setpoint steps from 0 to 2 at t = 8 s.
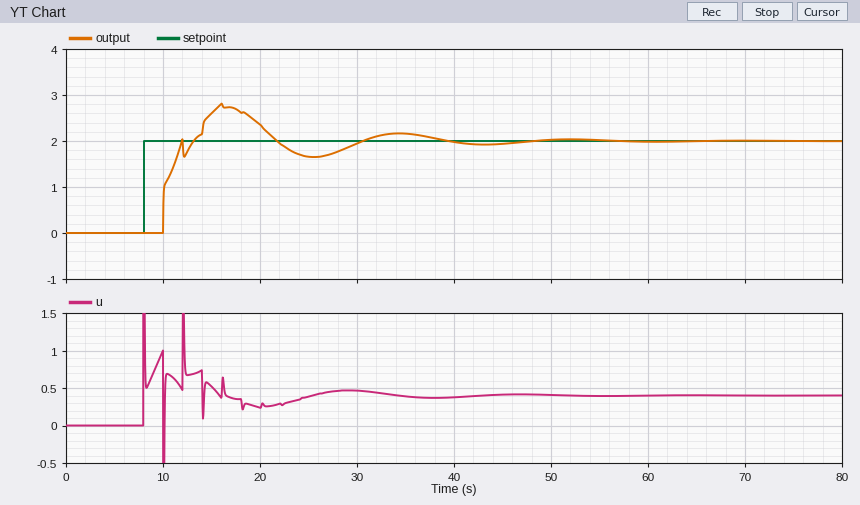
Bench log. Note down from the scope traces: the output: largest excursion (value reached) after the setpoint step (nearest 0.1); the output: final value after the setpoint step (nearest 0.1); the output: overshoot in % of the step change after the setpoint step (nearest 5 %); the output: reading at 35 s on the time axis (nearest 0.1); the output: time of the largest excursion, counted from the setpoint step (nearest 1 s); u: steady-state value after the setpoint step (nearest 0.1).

2.8
2.0
40 %
2.2
8 s
0.4
